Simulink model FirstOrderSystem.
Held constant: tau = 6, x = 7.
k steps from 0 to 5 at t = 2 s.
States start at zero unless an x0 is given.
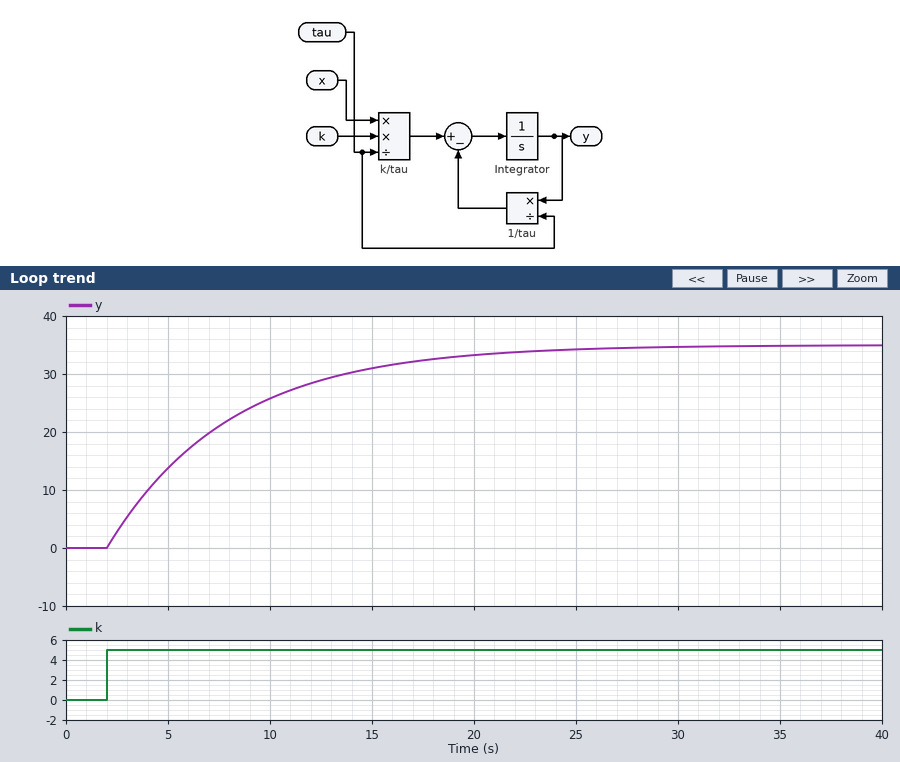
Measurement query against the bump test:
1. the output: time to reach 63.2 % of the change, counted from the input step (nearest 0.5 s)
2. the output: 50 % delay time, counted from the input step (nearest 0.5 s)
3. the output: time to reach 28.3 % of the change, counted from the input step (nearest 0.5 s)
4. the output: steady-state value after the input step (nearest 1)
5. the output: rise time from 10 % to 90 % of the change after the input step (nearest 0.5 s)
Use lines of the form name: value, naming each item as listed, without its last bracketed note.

the output: time to reach 63.2 % of the change, counted from the input step: 6.0 s
the output: 50 % delay time, counted from the input step: 4.0 s
the output: time to reach 28.3 % of the change, counted from the input step: 2.0 s
the output: steady-state value after the input step: 35
the output: rise time from 10 % to 90 % of the change after the input step: 13.0 s
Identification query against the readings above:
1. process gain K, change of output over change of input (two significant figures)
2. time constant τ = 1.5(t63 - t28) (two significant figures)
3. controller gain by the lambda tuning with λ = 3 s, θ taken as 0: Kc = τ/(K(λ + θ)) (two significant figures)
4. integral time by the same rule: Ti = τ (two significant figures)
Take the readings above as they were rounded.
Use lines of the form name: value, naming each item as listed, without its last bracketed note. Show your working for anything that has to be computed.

process gain K, change of output over change of input: (35 - 0) / 5 = 7.0
time constant τ = 1.5(t63 - t28): 1.5 × (6 - 2) = 6.0 s
controller gain by the lambda tuning with λ = 3 s, θ taken as 0: Kc = τ/(K(λ + θ)): 6 / (7 × (3 + 0)) = 0.29
integral time by the same rule: Ti = τ: 6.0 s
